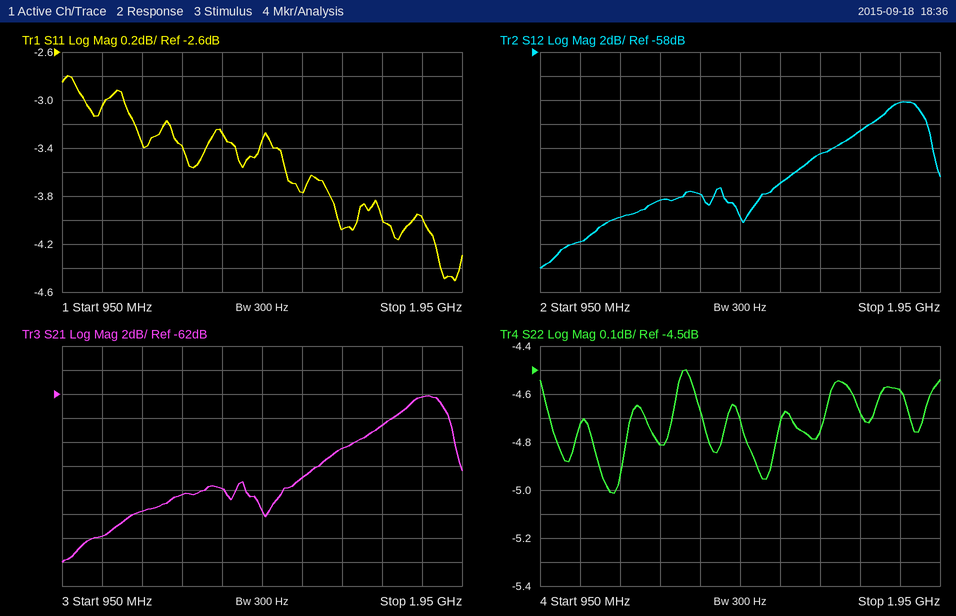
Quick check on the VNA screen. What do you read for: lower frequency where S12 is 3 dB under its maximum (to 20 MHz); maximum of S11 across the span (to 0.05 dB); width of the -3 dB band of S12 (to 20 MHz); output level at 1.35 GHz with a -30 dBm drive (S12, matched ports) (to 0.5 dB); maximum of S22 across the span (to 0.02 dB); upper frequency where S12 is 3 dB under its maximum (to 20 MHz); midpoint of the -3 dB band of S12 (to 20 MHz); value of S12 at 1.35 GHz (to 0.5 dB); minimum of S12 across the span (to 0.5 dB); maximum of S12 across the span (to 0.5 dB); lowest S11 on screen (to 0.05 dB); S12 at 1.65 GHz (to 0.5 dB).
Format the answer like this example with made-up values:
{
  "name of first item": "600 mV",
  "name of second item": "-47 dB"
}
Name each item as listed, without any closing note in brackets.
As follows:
{
  "lower frequency where S12 is 3 dB under its maximum": "1.72 GHz",
  "maximum of S11 across the span": "-2.80 dB",
  "width of the -3 dB band of S12": "200 MHz",
  "output level at 1.35 GHz with a -30 dBm drive (S12, matched ports)": "-100.0 dBm",
  "maximum of S22 across the span": "-4.50 dB",
  "upper frequency where S12 is 3 dB under its maximum": "1.92 GHz",
  "midpoint of the -3 dB band of S12": "1.82 GHz",
  "value of S12 at 1.35 GHz": "-70.0 dB",
  "minimum of S12 across the span": "-76.0 dB",
  "maximum of S12 across the span": "-62.0 dB",
  "lowest S11 on screen": "-4.50 dB",
  "S12 at 1.65 GHz": "-66.5 dB"
}
